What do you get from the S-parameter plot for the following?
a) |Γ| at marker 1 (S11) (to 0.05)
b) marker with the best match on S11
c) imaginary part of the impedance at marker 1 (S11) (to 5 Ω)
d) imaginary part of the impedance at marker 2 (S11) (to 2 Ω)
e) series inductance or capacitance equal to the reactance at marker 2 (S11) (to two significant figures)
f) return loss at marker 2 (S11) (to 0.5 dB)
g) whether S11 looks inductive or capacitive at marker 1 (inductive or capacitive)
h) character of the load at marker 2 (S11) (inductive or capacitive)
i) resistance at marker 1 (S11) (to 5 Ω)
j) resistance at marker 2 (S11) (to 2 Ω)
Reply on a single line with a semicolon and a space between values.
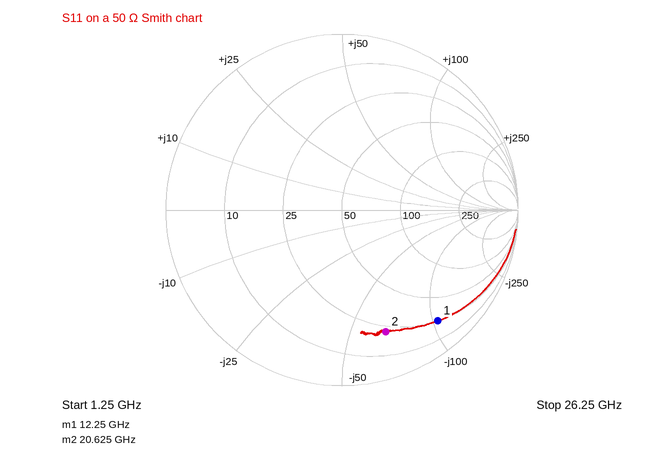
0.85; marker 2; -105 Ω; -66 Ω; 120 fF; 2.5 dB; capacitive; capacitive; 25 Ω; 22 Ω
